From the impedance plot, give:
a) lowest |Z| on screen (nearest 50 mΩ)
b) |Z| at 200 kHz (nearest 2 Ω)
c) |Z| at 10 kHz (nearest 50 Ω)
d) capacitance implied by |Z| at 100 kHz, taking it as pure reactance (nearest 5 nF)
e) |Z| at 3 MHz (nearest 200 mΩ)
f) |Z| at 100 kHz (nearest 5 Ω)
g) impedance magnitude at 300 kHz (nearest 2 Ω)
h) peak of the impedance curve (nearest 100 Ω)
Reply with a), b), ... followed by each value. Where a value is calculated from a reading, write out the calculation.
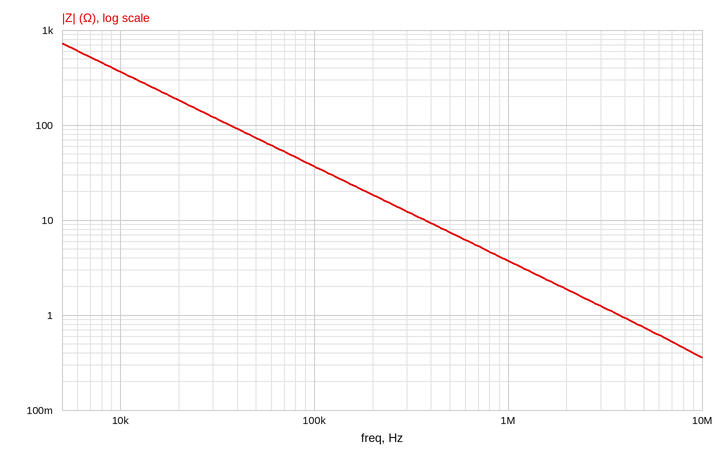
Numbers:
a) 350 mΩ
b) 18 Ω
c) 350 Ω
d) C = 1/(2π × 100 kHz × 35 Ω) ≈ 45 nF
e) 1.2 Ω
f) 35 Ω
g) 12 Ω
h) 700 Ω
